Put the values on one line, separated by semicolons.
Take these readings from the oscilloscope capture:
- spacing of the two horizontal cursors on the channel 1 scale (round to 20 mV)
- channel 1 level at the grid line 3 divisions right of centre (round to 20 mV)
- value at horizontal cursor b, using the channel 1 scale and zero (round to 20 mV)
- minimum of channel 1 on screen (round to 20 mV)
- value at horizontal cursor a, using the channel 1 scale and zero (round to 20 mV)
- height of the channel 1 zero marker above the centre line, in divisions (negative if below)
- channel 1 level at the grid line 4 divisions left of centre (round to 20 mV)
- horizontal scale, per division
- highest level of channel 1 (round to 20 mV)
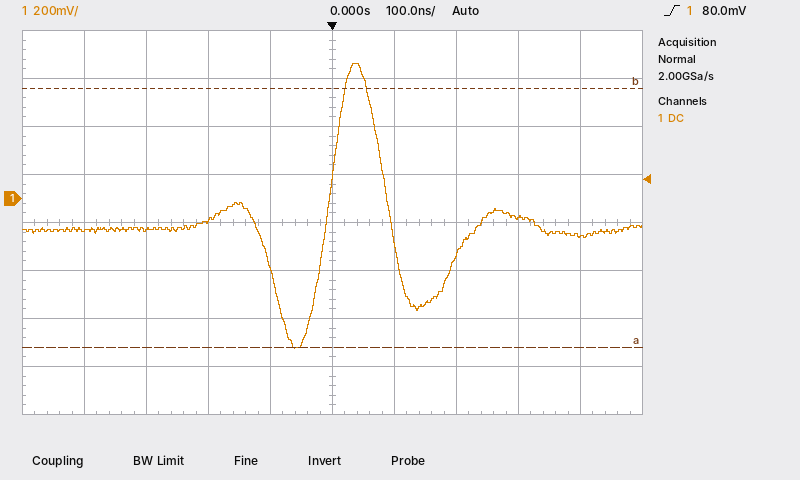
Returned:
1.08 V; -80 mV; 460 mV; -620 mV; -620 mV; +0.5 div; -140 mV; 100 ns; 560 mV
